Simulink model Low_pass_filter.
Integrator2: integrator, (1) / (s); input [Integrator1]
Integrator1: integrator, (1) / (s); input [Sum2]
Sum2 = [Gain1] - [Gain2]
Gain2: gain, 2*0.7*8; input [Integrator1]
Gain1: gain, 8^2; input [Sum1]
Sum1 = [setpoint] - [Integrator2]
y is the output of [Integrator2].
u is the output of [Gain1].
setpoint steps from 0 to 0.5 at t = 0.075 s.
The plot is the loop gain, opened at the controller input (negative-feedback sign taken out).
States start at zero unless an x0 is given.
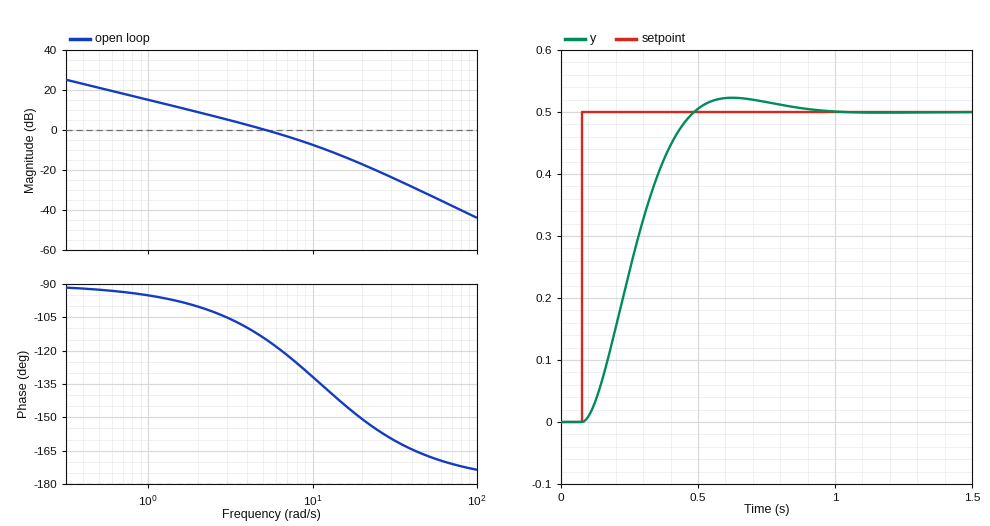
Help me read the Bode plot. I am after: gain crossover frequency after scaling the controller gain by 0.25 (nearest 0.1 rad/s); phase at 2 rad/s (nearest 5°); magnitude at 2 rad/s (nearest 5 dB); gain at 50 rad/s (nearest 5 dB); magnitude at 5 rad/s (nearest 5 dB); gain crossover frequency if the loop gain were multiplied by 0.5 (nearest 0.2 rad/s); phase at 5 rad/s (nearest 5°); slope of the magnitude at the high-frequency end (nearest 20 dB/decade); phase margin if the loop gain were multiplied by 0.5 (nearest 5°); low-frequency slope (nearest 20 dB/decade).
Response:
1.4 rad/s
-100°
10 dB
-30 dB
0 dB
2.8 rad/s
-115°
-40 dB/decade
75°
-20 dB/decade
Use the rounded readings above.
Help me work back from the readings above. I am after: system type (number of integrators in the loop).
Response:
1
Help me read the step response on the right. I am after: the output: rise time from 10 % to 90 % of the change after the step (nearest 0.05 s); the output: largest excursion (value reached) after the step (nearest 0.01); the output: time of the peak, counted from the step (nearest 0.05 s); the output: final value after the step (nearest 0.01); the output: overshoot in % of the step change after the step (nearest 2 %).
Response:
0.25 s
0.52
0.55 s
0.50
4 %
